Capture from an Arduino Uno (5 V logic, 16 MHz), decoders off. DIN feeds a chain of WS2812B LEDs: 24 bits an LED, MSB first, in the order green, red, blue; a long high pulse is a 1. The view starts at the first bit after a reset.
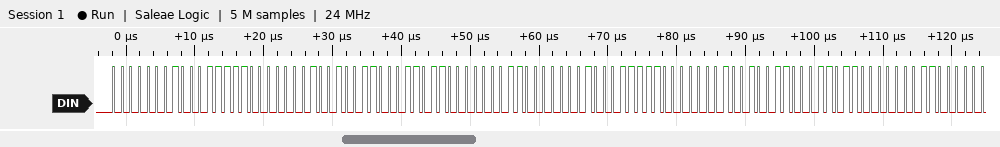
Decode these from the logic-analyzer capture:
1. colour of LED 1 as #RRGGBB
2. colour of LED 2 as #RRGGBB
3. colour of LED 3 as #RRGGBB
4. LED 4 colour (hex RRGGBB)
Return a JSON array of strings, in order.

["#1F0101", "#362603", "#1F0101", "#362603"]
